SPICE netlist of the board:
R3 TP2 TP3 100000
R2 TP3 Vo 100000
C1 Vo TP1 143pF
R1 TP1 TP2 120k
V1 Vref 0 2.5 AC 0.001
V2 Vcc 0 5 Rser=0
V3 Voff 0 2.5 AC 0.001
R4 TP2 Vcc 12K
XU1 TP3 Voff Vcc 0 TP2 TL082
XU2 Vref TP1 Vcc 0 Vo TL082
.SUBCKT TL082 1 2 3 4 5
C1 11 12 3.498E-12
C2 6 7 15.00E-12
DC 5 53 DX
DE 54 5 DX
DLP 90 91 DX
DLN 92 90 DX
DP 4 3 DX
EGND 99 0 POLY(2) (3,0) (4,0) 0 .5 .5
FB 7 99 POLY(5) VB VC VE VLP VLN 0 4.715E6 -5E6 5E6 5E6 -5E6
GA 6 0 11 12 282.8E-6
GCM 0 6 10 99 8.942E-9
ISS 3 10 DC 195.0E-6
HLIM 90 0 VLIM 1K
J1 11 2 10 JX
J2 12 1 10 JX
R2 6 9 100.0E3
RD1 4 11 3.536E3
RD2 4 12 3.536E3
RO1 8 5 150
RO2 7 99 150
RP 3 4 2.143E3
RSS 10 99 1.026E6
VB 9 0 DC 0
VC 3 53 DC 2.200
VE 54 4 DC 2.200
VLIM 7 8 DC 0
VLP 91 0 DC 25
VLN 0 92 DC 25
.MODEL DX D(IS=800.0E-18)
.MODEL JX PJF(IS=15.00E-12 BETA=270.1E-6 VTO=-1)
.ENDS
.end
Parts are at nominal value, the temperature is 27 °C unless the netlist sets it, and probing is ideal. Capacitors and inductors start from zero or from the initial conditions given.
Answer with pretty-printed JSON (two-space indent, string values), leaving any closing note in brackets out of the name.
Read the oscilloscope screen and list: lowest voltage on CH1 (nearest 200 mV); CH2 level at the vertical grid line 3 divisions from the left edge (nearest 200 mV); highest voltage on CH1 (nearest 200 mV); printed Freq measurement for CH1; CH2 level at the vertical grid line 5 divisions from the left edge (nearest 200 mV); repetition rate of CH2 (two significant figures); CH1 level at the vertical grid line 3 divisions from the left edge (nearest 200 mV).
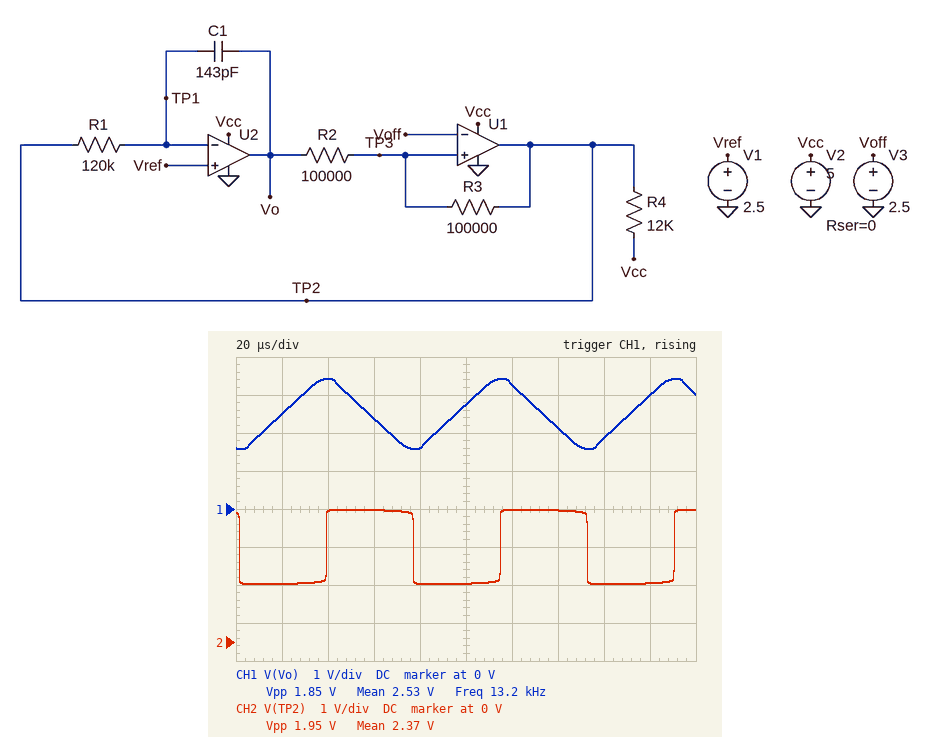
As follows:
{
  "lowest voltage on CH1": "1.6 V",
  "CH2 level at the vertical grid line 3 divisions from the left edge": "3.4 V",
  "highest voltage on CH1": "3.4 V",
  "printed Freq measurement for CH1": "13.2 kHz",
  "CH2 level at the vertical grid line 5 divisions from the left edge": "1.6 V",
  "repetition rate of CH2": "13 kHz",
  "CH1 level at the vertical grid line 3 divisions from the left edge": "2.4 V"
}
